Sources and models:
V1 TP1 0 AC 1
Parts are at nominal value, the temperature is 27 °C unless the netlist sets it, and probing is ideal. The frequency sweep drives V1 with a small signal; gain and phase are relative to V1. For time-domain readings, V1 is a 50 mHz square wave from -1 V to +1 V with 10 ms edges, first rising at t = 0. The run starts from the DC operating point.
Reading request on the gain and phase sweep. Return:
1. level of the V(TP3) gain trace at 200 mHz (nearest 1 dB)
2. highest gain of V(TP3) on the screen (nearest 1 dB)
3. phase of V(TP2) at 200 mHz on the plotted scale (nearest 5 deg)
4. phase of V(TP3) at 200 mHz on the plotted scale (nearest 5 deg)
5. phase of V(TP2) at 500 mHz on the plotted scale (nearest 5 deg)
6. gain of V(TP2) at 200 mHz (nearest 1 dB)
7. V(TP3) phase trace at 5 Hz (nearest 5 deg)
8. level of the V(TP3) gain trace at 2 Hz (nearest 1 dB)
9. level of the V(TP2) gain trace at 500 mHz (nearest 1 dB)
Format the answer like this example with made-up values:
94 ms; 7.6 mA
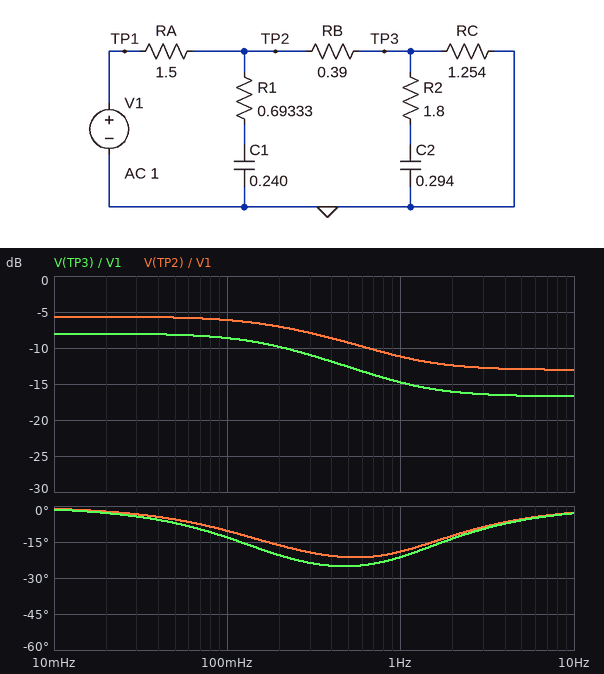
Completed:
-10 dB; -8 dB; -15 deg; -20 deg; -20 deg; -7 dB; -5 deg; -16 dB; -9 dB
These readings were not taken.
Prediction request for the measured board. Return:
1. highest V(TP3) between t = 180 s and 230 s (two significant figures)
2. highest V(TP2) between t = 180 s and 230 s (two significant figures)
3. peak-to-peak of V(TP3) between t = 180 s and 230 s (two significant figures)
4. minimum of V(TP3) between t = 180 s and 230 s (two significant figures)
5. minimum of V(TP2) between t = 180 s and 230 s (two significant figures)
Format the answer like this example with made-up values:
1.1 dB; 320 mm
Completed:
400 mV; 520 mV; 800 mV; -400 mV; -520 mV
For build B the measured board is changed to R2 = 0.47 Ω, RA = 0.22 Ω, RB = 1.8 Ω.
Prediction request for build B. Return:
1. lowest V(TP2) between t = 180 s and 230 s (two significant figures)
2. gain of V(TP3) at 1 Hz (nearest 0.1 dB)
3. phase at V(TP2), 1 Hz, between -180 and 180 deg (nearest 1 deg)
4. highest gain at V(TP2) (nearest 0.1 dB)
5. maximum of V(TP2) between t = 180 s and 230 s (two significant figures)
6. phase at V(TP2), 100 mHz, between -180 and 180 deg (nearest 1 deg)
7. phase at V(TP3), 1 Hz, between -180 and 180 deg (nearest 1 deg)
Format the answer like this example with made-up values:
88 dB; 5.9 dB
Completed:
-930 mV; -15.2 dB; -8 deg; -0.6 dB; 930 mV; -2 deg; -33 deg
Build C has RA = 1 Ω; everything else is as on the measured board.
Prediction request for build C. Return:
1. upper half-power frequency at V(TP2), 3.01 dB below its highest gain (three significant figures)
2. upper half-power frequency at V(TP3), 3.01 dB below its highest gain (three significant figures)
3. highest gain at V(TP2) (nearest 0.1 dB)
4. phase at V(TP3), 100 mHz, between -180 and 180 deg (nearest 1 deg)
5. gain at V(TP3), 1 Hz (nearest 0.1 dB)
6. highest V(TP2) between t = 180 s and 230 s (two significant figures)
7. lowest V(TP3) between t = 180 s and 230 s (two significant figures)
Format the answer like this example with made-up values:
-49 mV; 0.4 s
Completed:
519 mHz; 363 mHz; -4.1 dB; -11 deg; -12.3 dB; 620 mV; -470 mV
